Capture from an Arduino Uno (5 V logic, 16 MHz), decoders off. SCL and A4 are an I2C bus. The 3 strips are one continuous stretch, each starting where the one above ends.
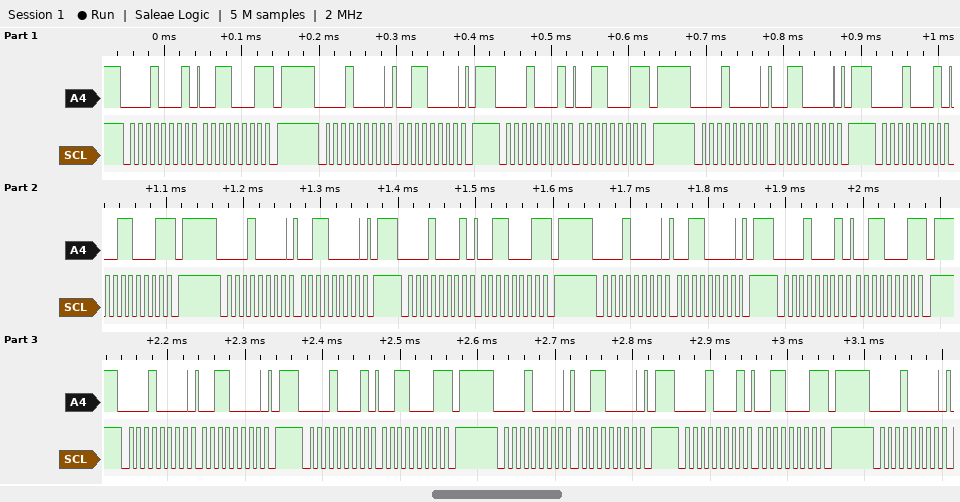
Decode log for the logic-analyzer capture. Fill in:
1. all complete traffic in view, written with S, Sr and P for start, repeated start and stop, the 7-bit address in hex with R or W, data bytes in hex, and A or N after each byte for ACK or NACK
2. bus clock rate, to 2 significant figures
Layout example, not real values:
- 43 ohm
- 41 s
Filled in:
- S 08R A 31 N P S 08W A 30 A P S 08R A 31 N P S 08W A 30 A P S 08R A 31 N P S 08W A 30 A P S 08R A 31 N P S 08W A 30 A P S 08R A 31 N P S 08W A 30 A P S 08R A 31 N P S 08W A 30 A P S 08R A 31 N P S 08W A
- 100 kHz
